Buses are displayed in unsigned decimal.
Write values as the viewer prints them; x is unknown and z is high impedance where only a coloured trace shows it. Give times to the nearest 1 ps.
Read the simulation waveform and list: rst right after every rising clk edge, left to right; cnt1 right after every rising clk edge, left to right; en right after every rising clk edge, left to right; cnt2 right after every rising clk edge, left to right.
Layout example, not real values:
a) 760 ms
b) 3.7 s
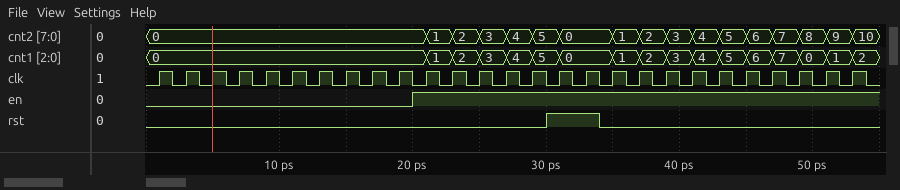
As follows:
a) 0 0 0 0 0 0 0 0 0 0 0 0 0 0 0 1 1 0 0 0 0 0 0 0 0 0 0
b) 0, 0, 0, 0, 0, 0, 0, 0, 0, 0, 1, 2, 3, 4, 5, 0, 0, 1, 2, 3, 4, 5, 6, 7, 0, 1, 2
c) 0 0 0 0 0 0 0 0 0 0 1 1 1 1 1 1 1 1 1 1 1 1 1 1 1 1 1
d) 0, 0, 0, 0, 0, 0, 0, 0, 0, 0, 1, 2, 3, 4, 5, 0, 0, 1, 2, 3, 4, 5, 6, 7, 8, 9, 10
